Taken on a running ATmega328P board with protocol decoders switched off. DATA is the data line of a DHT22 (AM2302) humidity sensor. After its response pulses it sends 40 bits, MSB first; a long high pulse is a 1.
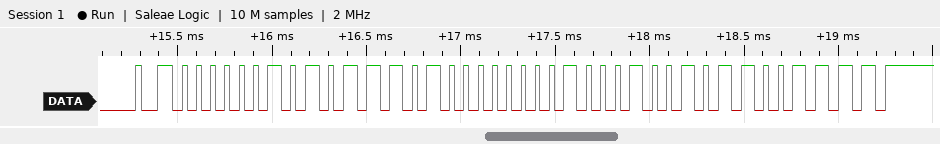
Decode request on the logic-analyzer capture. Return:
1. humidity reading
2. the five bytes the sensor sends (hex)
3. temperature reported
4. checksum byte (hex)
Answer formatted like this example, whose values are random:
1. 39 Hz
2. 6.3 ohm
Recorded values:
1. 69.8 %
2. 02 BA 01 12 CF
3. 27.4 °C
4. 0xCF
